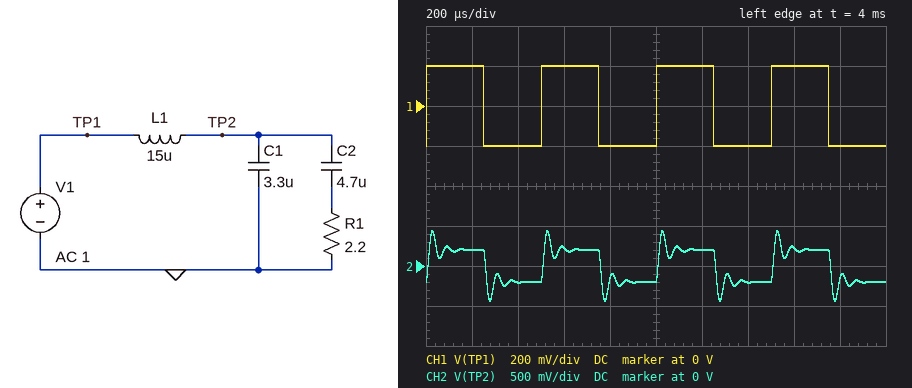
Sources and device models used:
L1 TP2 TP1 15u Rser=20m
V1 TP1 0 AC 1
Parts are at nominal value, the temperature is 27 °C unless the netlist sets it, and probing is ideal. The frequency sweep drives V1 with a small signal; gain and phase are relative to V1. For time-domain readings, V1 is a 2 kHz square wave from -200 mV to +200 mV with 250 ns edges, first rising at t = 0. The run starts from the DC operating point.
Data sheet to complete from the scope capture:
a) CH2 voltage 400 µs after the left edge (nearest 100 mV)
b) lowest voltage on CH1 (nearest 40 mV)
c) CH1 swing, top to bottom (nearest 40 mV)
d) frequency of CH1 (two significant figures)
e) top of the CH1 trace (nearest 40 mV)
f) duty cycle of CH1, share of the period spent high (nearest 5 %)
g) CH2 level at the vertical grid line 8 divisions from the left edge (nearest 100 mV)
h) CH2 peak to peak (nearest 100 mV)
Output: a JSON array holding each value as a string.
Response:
["-200 mV", "-200 mV", "400 mV", "2.0 kHz", "200 mV", "50 %", "200 mV", "900 mV"]
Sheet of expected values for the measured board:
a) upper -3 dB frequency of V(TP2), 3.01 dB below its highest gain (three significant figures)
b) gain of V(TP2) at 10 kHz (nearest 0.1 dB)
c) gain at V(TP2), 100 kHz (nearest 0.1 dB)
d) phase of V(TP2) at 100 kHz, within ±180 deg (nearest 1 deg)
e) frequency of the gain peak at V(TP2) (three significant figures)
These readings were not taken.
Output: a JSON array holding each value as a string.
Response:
["19.8 kHz", "4.1 dB", "-25.9 dB", "-168 deg", "15.7 kHz"]
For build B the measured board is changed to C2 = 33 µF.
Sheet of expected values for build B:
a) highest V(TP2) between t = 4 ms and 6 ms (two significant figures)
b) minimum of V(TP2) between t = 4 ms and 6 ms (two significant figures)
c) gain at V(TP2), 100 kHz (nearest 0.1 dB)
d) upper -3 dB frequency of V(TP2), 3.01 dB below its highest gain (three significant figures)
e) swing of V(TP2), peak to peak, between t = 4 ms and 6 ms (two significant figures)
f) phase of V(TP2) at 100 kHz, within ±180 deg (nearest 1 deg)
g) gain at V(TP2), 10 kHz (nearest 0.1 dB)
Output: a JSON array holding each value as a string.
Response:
["300 mV", "-300 mV", "-25.6 dB", "25.1 kHz", "600 mV", "-167 deg", "1.6 dB"]
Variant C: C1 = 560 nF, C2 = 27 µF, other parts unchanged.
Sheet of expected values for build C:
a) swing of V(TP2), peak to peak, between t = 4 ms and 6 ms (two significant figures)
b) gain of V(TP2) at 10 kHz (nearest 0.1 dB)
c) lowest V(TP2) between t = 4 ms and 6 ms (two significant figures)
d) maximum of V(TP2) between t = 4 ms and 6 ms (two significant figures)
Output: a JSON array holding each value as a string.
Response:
["460 mV", "0.4 dB", "-230 mV", "230 mV"]
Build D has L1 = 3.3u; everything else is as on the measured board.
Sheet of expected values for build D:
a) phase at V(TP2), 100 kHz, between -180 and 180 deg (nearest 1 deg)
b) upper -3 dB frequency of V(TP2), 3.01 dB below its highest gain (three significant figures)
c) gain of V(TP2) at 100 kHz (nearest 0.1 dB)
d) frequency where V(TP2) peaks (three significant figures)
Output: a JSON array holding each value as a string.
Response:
["-164 deg", "51.8 kHz", "-11.0 dB", "42.4 kHz"]
